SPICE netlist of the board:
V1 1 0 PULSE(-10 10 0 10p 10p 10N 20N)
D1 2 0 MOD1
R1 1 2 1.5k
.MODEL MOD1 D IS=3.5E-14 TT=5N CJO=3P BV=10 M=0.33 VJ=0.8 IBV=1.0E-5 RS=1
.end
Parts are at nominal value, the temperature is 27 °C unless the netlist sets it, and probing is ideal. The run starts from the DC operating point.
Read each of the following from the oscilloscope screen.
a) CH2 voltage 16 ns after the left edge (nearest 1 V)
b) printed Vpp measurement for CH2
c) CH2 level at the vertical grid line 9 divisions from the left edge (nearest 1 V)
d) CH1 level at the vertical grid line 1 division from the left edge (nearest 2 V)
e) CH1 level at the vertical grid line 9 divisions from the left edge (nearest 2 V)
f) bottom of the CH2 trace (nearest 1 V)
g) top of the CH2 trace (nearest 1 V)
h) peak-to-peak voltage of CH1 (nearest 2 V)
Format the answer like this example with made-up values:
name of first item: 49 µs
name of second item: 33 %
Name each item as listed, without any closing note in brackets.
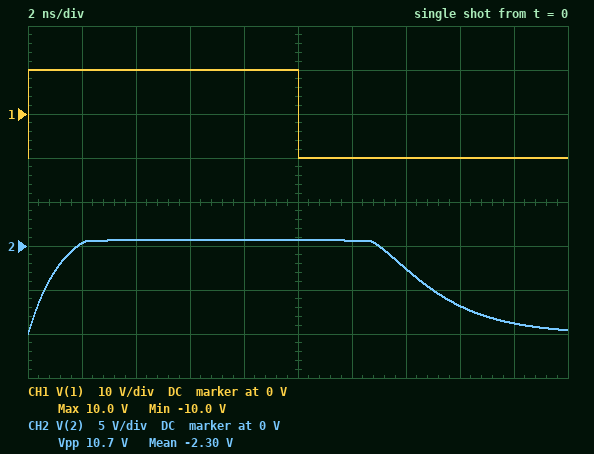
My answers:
CH2 voltage 16 ns after the left edge: -7 V
printed Vpp measurement for CH2: 10.7 V
CH2 level at the vertical grid line 9 divisions from the left edge: -9 V
CH1 level at the vertical grid line 1 division from the left edge: 10 V
CH1 level at the vertical grid line 9 divisions from the left edge: -10 V
bottom of the CH2 trace: -10 V
top of the CH2 trace: 1 V
peak-to-peak voltage of CH1: 20 V
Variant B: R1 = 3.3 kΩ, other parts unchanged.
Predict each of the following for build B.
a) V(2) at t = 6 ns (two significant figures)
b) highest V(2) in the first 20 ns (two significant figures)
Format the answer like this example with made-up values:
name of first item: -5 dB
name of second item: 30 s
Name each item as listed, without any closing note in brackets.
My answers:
V(2) at t = 6 ns: 610 mV
highest V(2) in the first 20 ns: 640 mV
